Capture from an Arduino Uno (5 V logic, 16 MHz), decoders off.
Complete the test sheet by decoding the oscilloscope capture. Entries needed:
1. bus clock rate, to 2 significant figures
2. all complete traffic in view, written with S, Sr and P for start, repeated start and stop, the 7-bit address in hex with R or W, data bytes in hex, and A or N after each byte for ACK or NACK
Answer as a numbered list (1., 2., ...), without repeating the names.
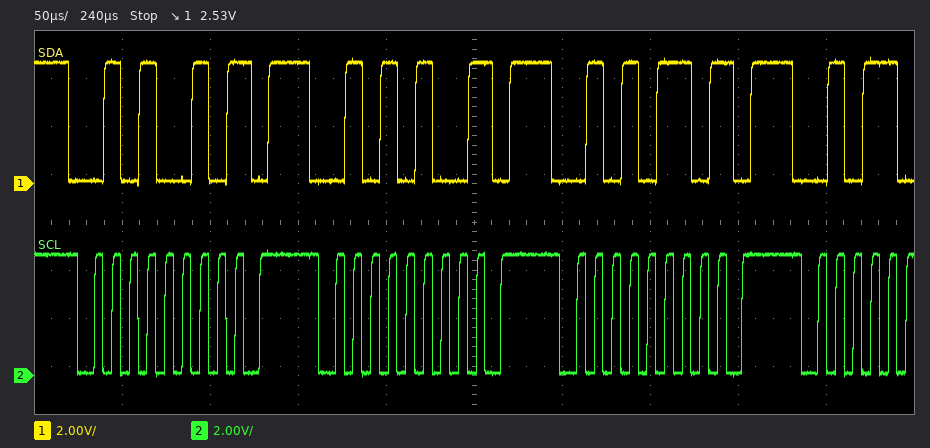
1. 100 kHz
2. S 29W N P S 2AW N P S 2BW N P
